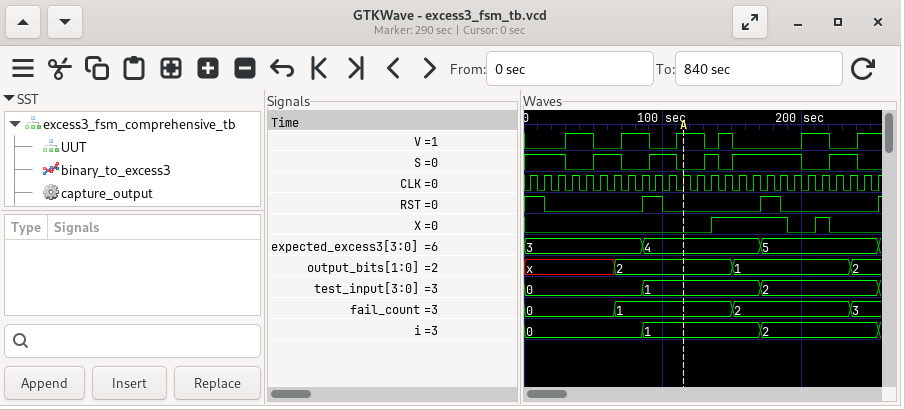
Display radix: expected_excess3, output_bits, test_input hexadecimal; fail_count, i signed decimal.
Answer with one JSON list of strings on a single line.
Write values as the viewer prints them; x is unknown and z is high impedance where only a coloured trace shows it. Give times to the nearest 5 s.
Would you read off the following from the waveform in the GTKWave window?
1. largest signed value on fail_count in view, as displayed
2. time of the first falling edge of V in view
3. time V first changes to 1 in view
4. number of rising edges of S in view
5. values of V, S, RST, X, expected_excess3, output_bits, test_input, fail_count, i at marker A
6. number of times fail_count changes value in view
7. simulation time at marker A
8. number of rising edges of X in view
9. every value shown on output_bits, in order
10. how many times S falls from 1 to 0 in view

["3", "50 s", "30 s", "5", "V=1, S=0, RST=0, X=0, expected_excess3=4, output_bits=2, test_input=1, fail_count=1, i=1", "3", "115 s", "2", "x, 2, 1, 2", "6"]
